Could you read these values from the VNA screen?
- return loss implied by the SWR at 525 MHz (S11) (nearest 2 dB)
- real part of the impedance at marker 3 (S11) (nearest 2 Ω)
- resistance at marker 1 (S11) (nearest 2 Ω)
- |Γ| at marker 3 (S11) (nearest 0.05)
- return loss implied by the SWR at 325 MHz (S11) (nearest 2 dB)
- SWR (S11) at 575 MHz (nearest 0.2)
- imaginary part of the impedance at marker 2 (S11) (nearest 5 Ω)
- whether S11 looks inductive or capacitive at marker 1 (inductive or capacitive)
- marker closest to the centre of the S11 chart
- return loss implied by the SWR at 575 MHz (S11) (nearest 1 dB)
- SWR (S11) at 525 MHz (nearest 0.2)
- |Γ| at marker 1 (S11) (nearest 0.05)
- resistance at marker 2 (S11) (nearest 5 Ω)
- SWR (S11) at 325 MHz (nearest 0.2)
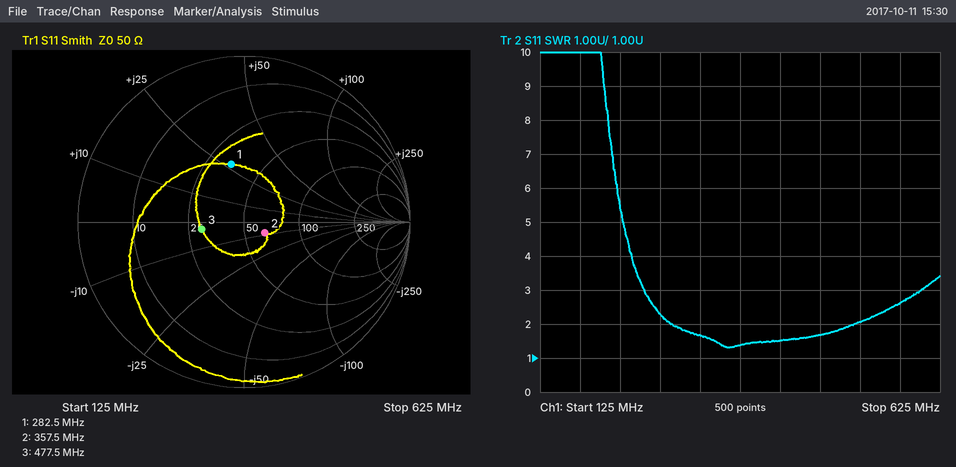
10 dB
30 Ω
34 Ω
0.25
12 dB
2.6
-10 Ω
inductive
marker 2
7 dB
2.0
0.35
65 Ω
1.6
